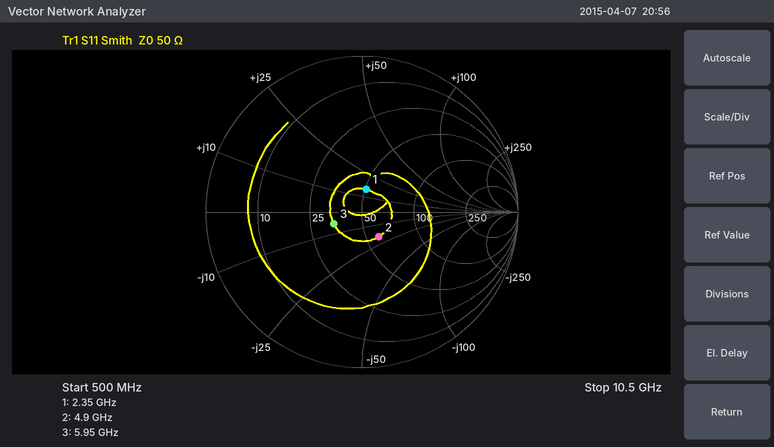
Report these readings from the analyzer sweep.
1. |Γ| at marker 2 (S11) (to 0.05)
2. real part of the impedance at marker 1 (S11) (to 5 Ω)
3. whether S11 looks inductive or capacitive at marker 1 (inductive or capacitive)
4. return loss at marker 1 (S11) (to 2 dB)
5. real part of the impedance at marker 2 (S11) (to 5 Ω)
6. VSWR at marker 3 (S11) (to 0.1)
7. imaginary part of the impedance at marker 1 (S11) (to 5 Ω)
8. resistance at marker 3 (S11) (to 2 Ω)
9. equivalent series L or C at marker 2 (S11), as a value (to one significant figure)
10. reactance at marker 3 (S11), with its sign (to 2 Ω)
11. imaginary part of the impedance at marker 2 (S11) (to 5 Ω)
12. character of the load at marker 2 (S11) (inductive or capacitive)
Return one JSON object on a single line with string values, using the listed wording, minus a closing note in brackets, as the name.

{"|Γ| at marker 2 (S11)": "0.20", "real part of the impedance at marker 1 (S11)": "50 Ω", "whether S11 looks inductive or capacitive at marker 1": "inductive", "return loss at marker 1 (S11)": "16 dB", "real part of the impedance at marker 2 (S11)": "60 Ω", "VSWR at marker 3 (S11)": "1.5", "imaginary part of the impedance at marker 1 (S11)": "+15 Ω", "resistance at marker 3 (S11)": "34 Ω", "equivalent series L or C at marker 2 (S11), as a value": "2 pF", "reactance at marker 3 (S11), with its sign": "-6 Ω", "imaginary part of the impedance at marker 2 (S11)": "-20 Ω", "character of the load at marker 2 (S11)": "capacitive"}
